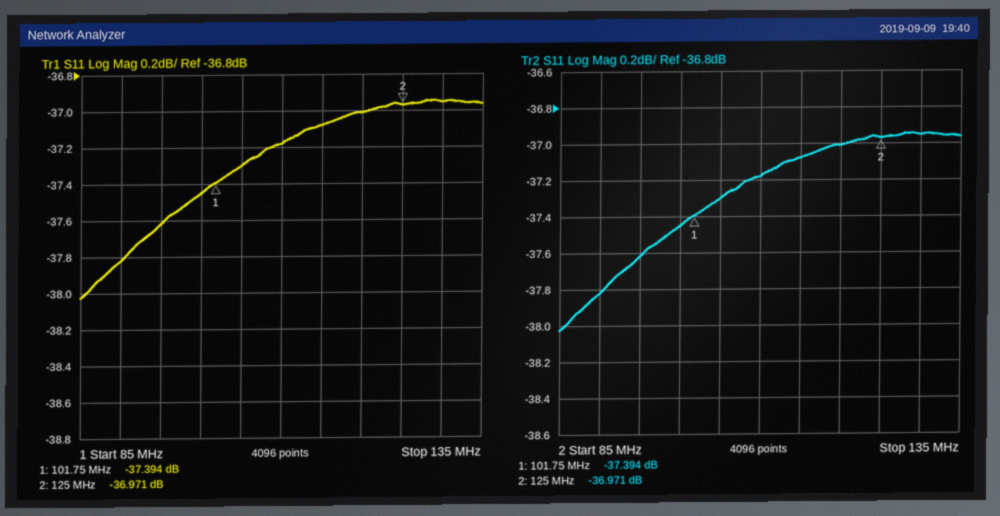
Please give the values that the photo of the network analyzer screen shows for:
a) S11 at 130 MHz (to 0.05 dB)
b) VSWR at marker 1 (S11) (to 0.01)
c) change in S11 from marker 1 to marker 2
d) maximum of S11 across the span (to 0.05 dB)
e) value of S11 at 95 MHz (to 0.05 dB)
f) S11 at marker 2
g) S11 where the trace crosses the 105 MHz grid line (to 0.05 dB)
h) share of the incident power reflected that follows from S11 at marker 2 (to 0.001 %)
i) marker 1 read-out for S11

-36.95 dB
1.03
0.423 dB
-36.95 dB
-37.60 dB
-36.971 dB
-37.30 dB
0.020 %
-37.394 dB
